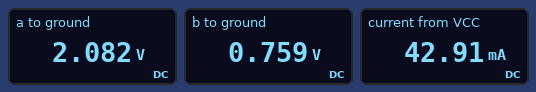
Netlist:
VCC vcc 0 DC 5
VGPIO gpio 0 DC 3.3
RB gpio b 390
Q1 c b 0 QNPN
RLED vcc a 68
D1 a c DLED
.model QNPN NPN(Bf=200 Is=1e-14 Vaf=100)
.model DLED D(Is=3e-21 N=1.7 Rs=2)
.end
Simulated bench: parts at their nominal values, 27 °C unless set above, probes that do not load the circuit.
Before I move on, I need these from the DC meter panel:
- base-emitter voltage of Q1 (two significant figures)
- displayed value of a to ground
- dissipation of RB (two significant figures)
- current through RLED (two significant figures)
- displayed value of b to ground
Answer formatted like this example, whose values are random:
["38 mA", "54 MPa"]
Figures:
["760 mV", "2.082 V", "17 mW", "43 mA", "0.759 V"]
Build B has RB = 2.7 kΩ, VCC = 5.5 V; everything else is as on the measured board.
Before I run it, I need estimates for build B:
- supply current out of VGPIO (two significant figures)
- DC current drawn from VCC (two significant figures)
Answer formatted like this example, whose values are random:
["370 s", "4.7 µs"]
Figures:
["940 µA", "49 mA"]
